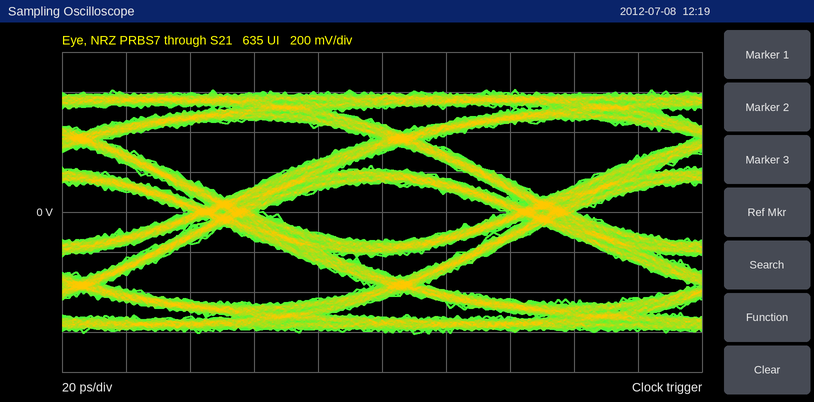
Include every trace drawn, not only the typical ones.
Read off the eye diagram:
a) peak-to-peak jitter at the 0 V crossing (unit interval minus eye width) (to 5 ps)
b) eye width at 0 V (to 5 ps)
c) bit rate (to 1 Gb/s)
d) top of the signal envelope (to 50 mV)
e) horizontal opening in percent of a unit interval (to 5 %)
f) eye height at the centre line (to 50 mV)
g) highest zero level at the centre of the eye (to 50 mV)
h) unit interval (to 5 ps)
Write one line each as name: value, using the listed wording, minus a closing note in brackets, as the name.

peak-to-peak jitter at the 0 V crossing (unit interval minus eye width): 25 ps
eye width at 0 V: 75 ps
bit rate: 10 Gb/s
top of the signal envelope: 600 mV
horizontal opening in percent of a unit interval: 75 %
eye height at the centre line: 300 mV
highest zero level at the centre of the eye: -150 mV
unit interval: 100 ps
